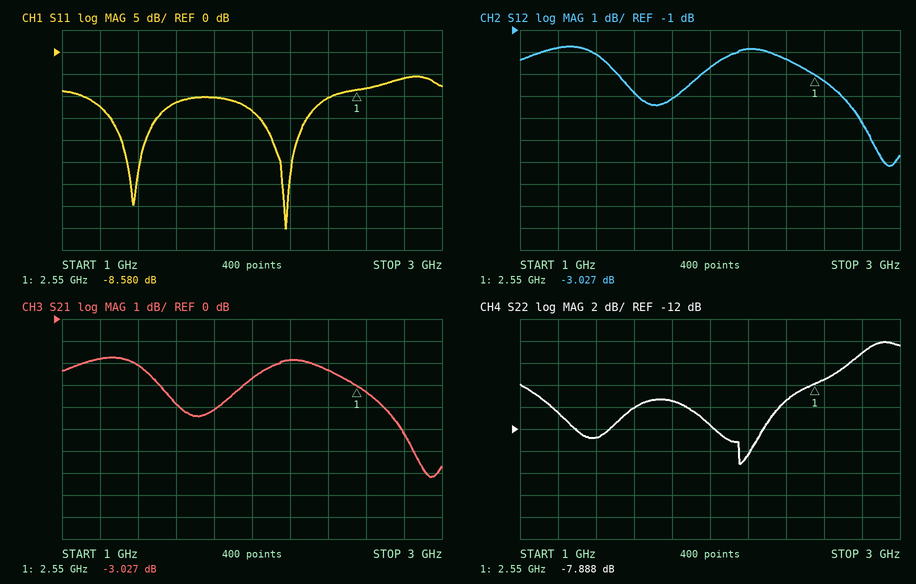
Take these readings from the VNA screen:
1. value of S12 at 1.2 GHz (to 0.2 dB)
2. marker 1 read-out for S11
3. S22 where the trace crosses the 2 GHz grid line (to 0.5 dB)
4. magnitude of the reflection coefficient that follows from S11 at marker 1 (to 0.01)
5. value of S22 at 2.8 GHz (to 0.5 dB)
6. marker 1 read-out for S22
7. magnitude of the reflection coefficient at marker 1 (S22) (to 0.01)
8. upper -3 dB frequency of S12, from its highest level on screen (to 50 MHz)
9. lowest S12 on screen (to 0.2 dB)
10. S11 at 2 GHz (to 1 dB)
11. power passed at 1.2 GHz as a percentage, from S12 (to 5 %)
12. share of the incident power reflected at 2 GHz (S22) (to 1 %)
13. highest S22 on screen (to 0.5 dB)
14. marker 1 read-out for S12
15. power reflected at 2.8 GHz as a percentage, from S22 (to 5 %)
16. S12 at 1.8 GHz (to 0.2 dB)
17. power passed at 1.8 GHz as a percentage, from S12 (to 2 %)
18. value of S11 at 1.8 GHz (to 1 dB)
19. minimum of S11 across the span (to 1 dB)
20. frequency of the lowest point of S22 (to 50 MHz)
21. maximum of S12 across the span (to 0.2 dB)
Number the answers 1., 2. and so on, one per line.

1. -1.8 dB
2. -8.580 dB
3. -11.5 dB
4. 0.37
5. -5.0 dB
6. -7.888 dB
7. 0.40
8. 2.75 GHz
9. -7.2 dB
10. -13 dB
11. 65 %
12. 7 %
13. -4.0 dB
14. -3.027 dB
15. 30 %
16. -4.2 dB
17. 38 %
18. -10 dB
19. -40 dB
20. 2.15 GHz
21. -1.8 dB
